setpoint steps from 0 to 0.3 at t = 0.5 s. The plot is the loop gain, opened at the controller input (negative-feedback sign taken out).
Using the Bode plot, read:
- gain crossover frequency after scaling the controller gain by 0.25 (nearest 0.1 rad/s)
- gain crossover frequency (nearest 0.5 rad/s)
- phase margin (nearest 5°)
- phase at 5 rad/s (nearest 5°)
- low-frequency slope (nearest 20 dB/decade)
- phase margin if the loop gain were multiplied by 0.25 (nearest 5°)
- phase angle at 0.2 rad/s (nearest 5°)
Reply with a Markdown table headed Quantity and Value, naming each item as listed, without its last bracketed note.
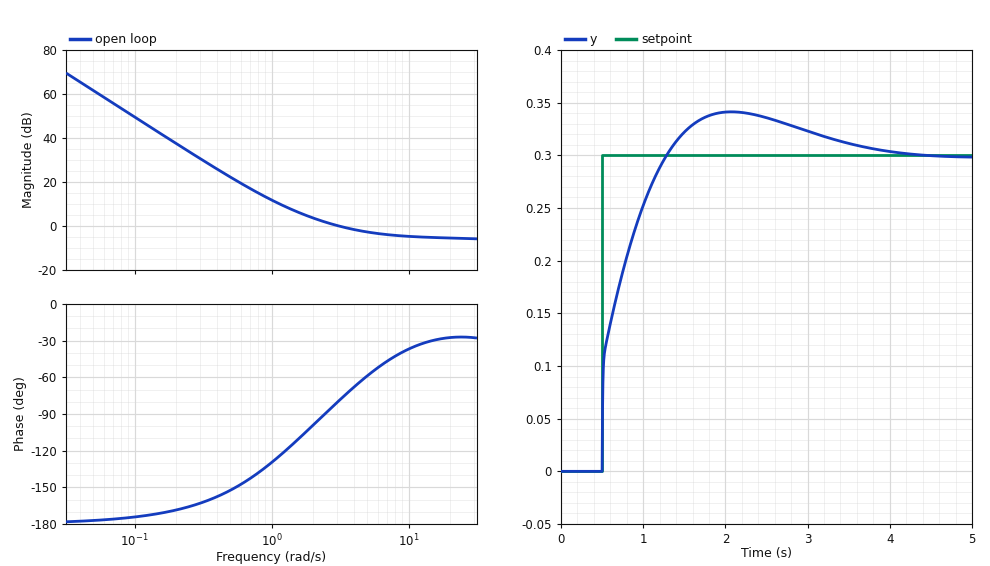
| Quantity | Value |
|---|---|
| gain crossover frequency after scaling the controller gain by 0.25 | 1.0 rad/s |
| gain crossover frequency | 3.0 rad/s |
| phase margin | 100° |
| phase at 5 rad/s | -60° |
| low-frequency slope | -40 dB/decade |
| phase margin if the loop gain were multiplied by 0.25 | 50° |
| phase angle at 0.2 rad/s | -170° |
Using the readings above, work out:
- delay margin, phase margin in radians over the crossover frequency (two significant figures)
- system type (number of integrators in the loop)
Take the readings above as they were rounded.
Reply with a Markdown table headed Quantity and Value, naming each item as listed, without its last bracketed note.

| Quantity | Value |
|---|---|
| delay margin, phase margin in radians over the crossover frequency | 0.58 s |
| system type | 2 |
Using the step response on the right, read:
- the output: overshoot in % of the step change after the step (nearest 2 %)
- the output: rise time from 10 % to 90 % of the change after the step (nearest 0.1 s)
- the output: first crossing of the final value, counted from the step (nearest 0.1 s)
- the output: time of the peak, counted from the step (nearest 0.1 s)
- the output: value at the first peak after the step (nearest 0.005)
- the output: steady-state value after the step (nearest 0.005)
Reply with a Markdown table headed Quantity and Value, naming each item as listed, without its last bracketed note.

| Quantity | Value |
|---|---|
| the output: overshoot in % of the step change after the step | 14 % |
| the output: rise time from 10 % to 90 % of the change after the step | 0.6 s |
| the output: first crossing of the final value, counted from the step | 0.8 s |
| the output: time of the peak, counted from the step | 1.6 s |
| the output: value at the first peak after the step | 0.340 |
| the output: steady-state value after the step | 0.300 |
